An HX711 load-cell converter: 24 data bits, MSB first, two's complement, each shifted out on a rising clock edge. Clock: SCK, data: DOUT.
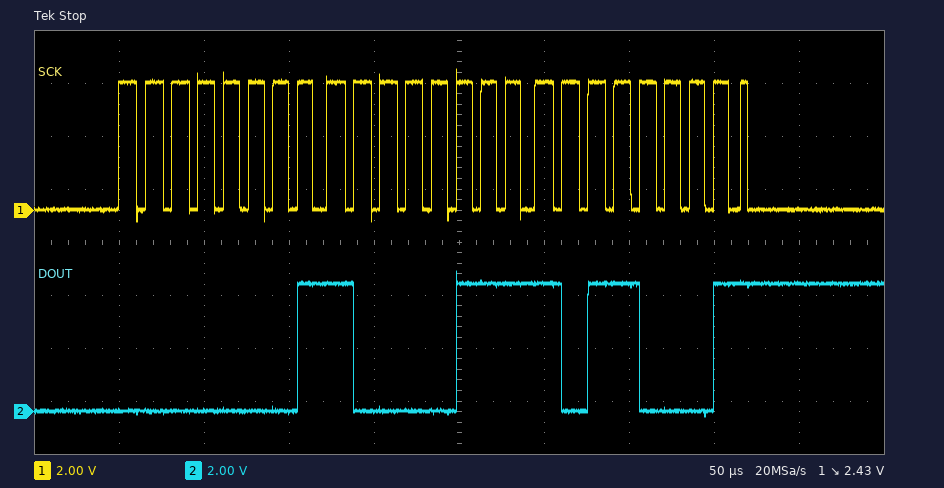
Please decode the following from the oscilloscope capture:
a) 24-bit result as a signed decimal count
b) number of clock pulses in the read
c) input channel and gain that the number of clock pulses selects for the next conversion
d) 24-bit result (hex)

100273
25
channel A, gain 128
0x0187B1
